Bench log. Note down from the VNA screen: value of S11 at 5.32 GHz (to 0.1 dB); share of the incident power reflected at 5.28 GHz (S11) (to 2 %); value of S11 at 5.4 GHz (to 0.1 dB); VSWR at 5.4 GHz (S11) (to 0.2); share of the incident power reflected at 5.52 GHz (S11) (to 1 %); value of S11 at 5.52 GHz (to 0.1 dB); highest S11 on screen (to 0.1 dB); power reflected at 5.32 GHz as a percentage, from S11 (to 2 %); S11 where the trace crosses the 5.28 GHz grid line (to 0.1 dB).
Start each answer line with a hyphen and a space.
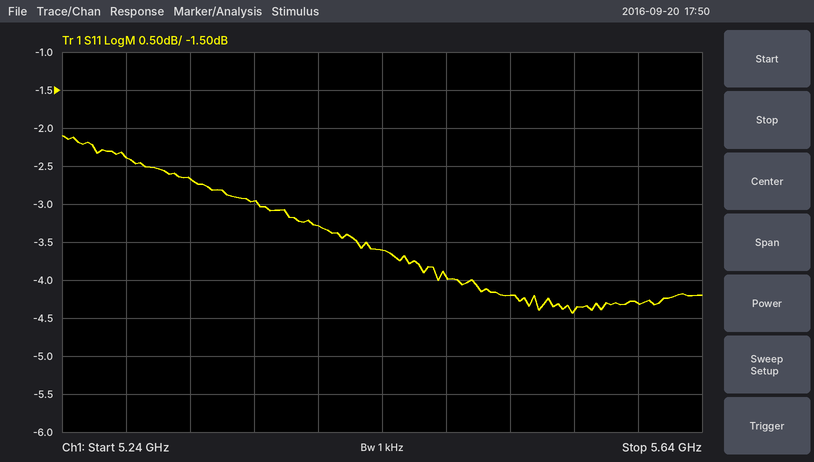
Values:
- -2.7 dB
- 58 %
- -3.3 dB
- 5.4
- 38 %
- -4.2 dB
- -2.1 dB
- 54 %
- -2.4 dB
